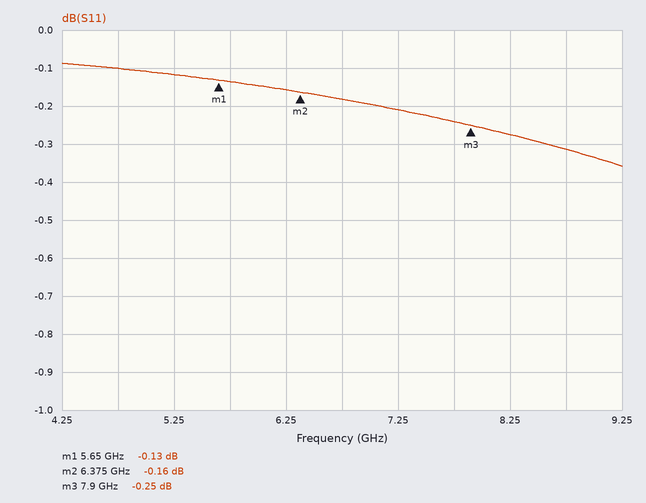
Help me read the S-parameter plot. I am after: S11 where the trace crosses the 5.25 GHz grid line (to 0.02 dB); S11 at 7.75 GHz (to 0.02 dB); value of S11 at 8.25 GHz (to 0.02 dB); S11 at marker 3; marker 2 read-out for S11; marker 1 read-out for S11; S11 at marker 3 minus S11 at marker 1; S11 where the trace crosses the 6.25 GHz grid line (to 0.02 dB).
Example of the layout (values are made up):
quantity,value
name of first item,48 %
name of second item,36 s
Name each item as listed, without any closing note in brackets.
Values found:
quantity,value
S11 where the trace crosses the 5.25 GHz grid line,-0.12 dB
S11 at 7.75 GHz,-0.24 dB
value of S11 at 8.25 GHz,-0.28 dB
S11 at marker 3,-0.25 dB
marker 2 read-out for S11,-0.16 dB
marker 1 read-out for S11,-0.13 dB
S11 at marker 3 minus S11 at marker 1,-0.12 dB
S11 where the trace crosses the 6.25 GHz grid line,-0.16 dB
